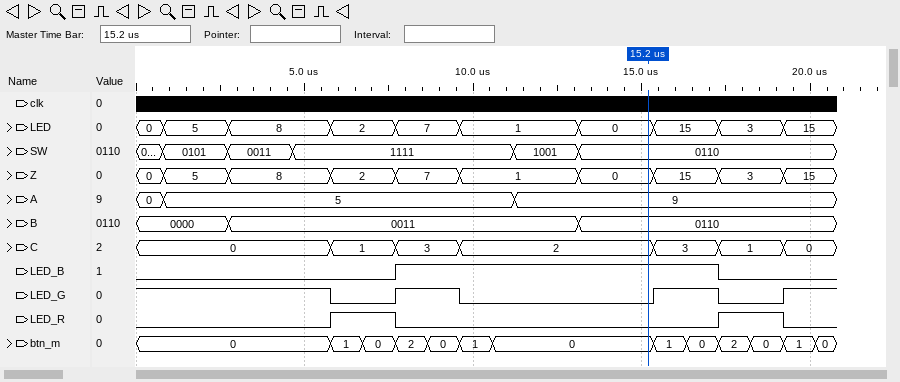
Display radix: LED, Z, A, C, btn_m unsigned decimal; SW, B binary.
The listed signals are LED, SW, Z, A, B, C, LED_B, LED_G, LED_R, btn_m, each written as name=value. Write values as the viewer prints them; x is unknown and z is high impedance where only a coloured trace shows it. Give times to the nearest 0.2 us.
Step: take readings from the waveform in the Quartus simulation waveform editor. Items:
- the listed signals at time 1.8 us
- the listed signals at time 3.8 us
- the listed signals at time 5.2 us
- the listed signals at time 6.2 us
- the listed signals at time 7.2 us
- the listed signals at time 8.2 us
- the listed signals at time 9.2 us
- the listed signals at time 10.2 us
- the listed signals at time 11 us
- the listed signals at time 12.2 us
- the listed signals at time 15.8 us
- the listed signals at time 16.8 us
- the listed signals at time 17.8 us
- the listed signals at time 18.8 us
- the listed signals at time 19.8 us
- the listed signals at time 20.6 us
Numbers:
LED=5, SW=0101, Z=5, A=5, B=0000, C=0, LED_B=0, LED_G=1, LED_R=0, btn_m=0
LED=8, SW=0011, Z=8, A=5, B=0011, C=0, LED_B=0, LED_G=1, LED_R=0, btn_m=0
LED=8, SW=1111, Z=8, A=5, B=0011, C=0, LED_B=0, LED_G=1, LED_R=0, btn_m=0
LED=2, SW=1111, Z=2, A=5, B=0011, C=1, LED_B=0, LED_G=0, LED_R=1, btn_m=1
LED=2, SW=1111, Z=2, A=5, B=0011, C=1, LED_B=0, LED_G=0, LED_R=1, btn_m=0
LED=7, SW=1111, Z=7, A=5, B=0011, C=3, LED_B=1, LED_G=1, LED_R=0, btn_m=2
LED=7, SW=1111, Z=7, A=5, B=0011, C=3, LED_B=1, LED_G=1, LED_R=0, btn_m=0
LED=1, SW=1111, Z=1, A=5, B=0011, C=2, LED_B=1, LED_G=0, LED_R=0, btn_m=1
LED=1, SW=1111, Z=1, A=5, B=0011, C=2, LED_B=1, LED_G=0, LED_R=0, btn_m=0
LED=1, SW=1001, Z=1, A=9, B=0011, C=2, LED_B=1, LED_G=0, LED_R=0, btn_m=0
LED=15, SW=0110, Z=15, A=9, B=0110, C=3, LED_B=1, LED_G=1, LED_R=0, btn_m=1
LED=15, SW=0110, Z=15, A=9, B=0110, C=3, LED_B=1, LED_G=1, LED_R=0, btn_m=0
LED=3, SW=0110, Z=3, A=9, B=0110, C=1, LED_B=0, LED_G=0, LED_R=1, btn_m=2
LED=3, SW=0110, Z=3, A=9, B=0110, C=1, LED_B=0, LED_G=0, LED_R=1, btn_m=0
LED=15, SW=0110, Z=15, A=9, B=0110, C=0, LED_B=0, LED_G=1, LED_R=0, btn_m=1
LED=15, SW=0110, Z=15, A=9, B=0110, C=0, LED_B=0, LED_G=1, LED_R=0, btn_m=0
